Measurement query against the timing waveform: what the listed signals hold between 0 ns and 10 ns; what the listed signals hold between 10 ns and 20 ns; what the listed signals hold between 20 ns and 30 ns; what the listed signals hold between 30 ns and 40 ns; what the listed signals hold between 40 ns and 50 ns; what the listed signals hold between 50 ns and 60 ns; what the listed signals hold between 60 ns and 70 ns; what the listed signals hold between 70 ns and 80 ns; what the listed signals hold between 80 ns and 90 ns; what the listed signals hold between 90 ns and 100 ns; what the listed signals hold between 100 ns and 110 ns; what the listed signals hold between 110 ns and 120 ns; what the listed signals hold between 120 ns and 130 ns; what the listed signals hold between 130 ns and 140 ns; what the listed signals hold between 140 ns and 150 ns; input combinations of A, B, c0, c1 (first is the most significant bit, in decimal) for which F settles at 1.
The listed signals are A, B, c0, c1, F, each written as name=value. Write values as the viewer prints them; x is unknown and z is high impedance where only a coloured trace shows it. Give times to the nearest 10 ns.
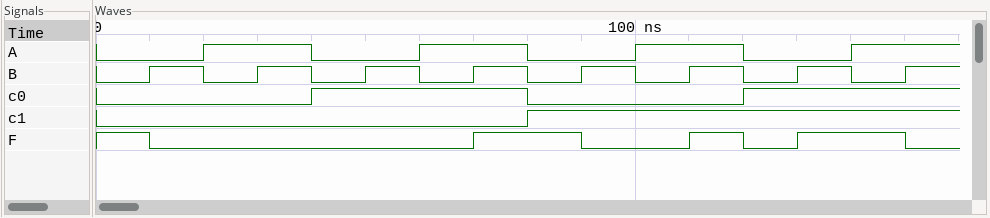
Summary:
A=0, B=0, c0=0, c1=0, F=1
A=0, B=1, c0=0, c1=0, F=0
A=1, B=0, c0=0, c1=0, F=0
A=1, B=1, c0=0, c1=0, F=0
A=0, B=0, c0=1, c1=0, F=0
A=0, B=1, c0=1, c1=0, F=0
A=1, B=0, c0=1, c1=0, F=0
A=1, B=1, c0=1, c1=0, F=1
A=0, B=0, c0=0, c1=1, F=1
A=0, B=1, c0=0, c1=1, F=0
A=1, B=0, c0=0, c1=1, F=0
A=1, B=1, c0=0, c1=1, F=1
A=0, B=0, c0=1, c1=1, F=0
A=0, B=1, c0=1, c1=1, F=1
A=1, B=0, c0=1, c1=1, F=1
0, 1, 7, 11, 13, 14
